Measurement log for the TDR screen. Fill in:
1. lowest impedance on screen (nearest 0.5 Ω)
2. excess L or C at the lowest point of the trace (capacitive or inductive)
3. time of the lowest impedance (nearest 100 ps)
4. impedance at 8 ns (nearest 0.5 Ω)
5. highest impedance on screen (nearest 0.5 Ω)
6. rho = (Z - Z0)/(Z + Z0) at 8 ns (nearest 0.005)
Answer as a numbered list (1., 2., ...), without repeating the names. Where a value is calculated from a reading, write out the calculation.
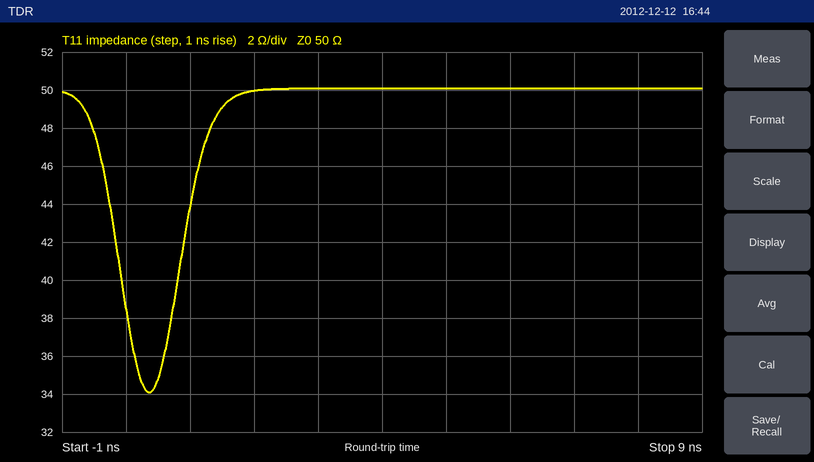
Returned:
1. 34.0 Ω
2. capacitive
3. 400 ps
4. 50.0 Ω
5. 50.0 Ω
6. (50 − 50)/(50 + 50) ≈ 0.000
